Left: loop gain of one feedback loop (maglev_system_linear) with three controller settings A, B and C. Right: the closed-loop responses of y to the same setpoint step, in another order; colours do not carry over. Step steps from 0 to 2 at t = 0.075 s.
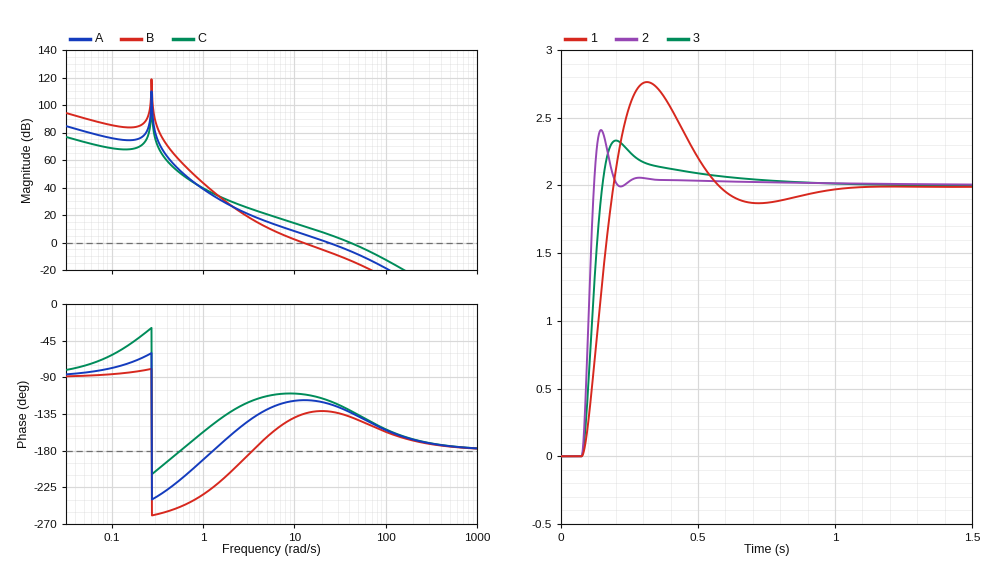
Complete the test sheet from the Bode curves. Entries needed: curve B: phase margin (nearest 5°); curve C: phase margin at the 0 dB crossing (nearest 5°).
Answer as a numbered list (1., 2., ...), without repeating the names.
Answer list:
1. 45°
2. 50°
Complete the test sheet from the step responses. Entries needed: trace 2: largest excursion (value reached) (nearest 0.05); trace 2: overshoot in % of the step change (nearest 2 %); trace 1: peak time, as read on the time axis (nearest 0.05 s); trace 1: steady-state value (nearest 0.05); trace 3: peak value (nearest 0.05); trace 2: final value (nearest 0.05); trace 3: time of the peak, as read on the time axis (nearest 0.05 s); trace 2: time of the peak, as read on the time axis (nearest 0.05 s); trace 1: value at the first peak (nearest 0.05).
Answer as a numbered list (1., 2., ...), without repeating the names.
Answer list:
1. 2.40
2. 20 %
3. 0.30 s
4. 2.00
5. 2.35
6. 2.00
7. 0.20 s
8. 0.15 s
9. 2.75
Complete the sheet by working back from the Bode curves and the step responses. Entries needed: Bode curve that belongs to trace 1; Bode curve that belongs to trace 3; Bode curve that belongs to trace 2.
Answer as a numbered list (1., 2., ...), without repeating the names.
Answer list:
1. B
2. A
3. C
